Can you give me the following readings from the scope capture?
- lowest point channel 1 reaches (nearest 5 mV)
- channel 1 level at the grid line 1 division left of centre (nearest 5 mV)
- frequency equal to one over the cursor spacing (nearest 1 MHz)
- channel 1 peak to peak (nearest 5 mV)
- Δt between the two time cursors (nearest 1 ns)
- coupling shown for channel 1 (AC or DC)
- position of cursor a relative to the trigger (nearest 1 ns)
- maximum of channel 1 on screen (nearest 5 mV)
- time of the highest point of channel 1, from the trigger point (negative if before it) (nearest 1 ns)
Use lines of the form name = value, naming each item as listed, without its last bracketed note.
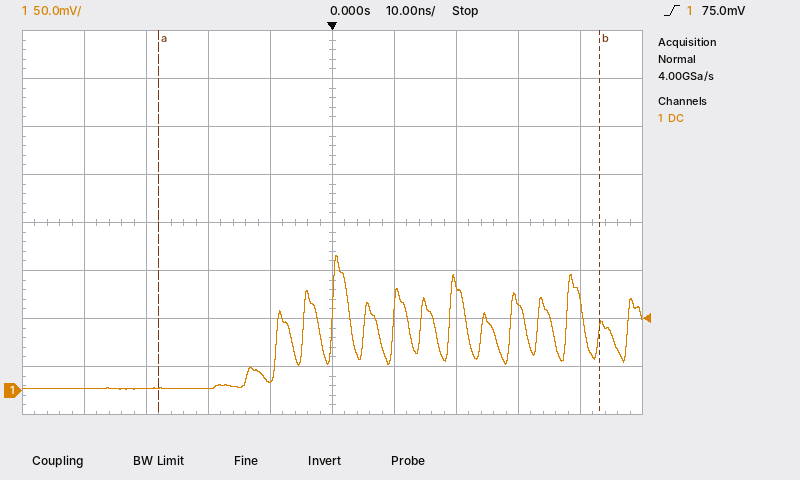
lowest point channel 1 reaches = 0 mV
channel 1 level at the grid line 1 division left of centre = 10 mV
frequency equal to one over the cursor spacing = 14 MHz
channel 1 peak to peak = 140 mV
Δt between the two time cursors = 71 ns
coupling shown for channel 1 = DC
position of cursor a relative to the trigger = -28 ns
maximum of channel 1 on screen = 140 mV
time of the highest point of channel 1, from the trigger point (negative if before it) = +1 ns
